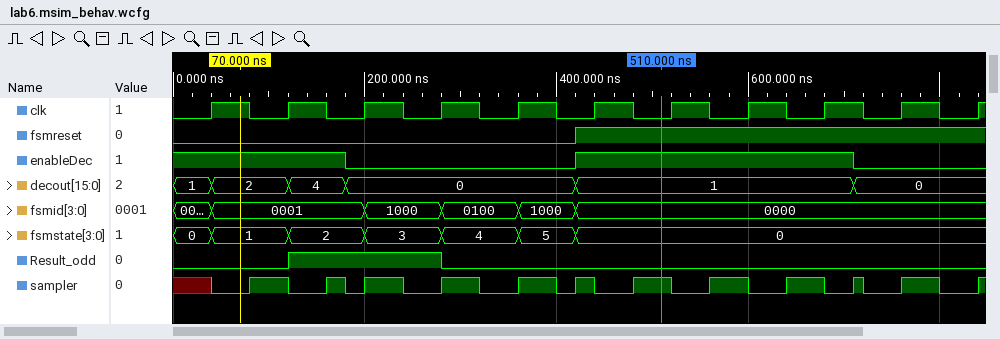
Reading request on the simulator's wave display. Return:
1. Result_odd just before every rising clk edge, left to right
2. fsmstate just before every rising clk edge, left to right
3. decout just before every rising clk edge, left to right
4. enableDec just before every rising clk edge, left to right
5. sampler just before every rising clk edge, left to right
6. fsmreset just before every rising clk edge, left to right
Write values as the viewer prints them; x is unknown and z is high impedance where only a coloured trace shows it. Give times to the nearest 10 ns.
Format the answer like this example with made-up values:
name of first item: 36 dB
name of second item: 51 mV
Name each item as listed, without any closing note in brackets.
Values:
Result_odd just before every rising clk edge, left to right: 0 0 1 1 0 0 0 0 0 0 0
fsmstate just before every rising clk edge, left to right: 0, 1, 2, 3, 4, 0, 0, 0, 0, 0, 0
decout just before every rising clk edge, left to right: 1, 2, 0, 0, 0, 1, 1, 1, 1, 0, 0
enableDec just before every rising clk edge, left to right: 1 1 0 0 0 1 1 1 1 0 0
sampler just before every rising clk edge, left to right: x 1 0 0 0 1 1 1 1 0 0
fsmreset just before every rising clk edge, left to right: 0 0 0 0 0 1 1 1 1 1 1
